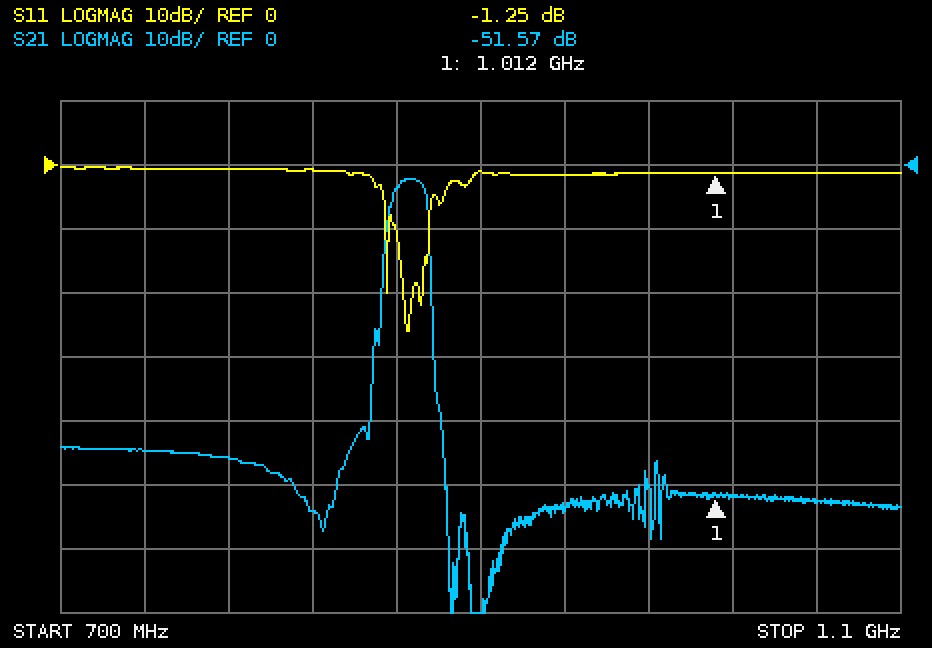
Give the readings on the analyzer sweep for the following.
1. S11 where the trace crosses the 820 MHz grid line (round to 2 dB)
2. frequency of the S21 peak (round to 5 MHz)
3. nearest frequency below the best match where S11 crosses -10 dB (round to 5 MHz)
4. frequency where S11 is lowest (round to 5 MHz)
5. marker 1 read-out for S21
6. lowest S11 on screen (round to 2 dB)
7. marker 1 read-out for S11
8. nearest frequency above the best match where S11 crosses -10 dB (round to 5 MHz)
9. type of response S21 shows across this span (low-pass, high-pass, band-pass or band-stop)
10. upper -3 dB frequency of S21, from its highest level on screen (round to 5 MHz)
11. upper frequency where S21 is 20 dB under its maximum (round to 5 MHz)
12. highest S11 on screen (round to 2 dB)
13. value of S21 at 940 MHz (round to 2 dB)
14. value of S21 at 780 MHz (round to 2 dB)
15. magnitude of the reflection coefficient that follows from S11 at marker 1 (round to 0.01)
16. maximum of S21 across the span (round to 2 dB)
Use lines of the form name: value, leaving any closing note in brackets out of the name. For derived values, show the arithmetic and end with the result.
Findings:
S11 where the trace crosses the 820 MHz grid line: 0 dB
frequency of the S21 peak: 865 MHz
nearest frequency below the best match where S11 crosses -10 dB: 860 MHz
frequency where S11 is lowest: 865 MHz
marker 1 read-out for S21: -51.57 dB
lowest S11 on screen: -26 dB
marker 1 read-out for S11: -1.25 dB
nearest frequency above the best match where S11 crosses -10 dB: 875 MHz
type of response S21 shows across this span: band-pass
upper -3 dB frequency of S21, from its highest level on screen: 875 MHz
upper frequency where S21 is 20 dB under its maximum: 875 MHz
highest S11 on screen: 0 dB
value of S21 at 940 MHz: -54 dB
value of S21 at 780 MHz: -46 dB
magnitude of the reflection coefficient that follows from S11 at marker 1: 10^(-1.25/20) ≈ 0.87
maximum of S21 across the span: -2 dB
